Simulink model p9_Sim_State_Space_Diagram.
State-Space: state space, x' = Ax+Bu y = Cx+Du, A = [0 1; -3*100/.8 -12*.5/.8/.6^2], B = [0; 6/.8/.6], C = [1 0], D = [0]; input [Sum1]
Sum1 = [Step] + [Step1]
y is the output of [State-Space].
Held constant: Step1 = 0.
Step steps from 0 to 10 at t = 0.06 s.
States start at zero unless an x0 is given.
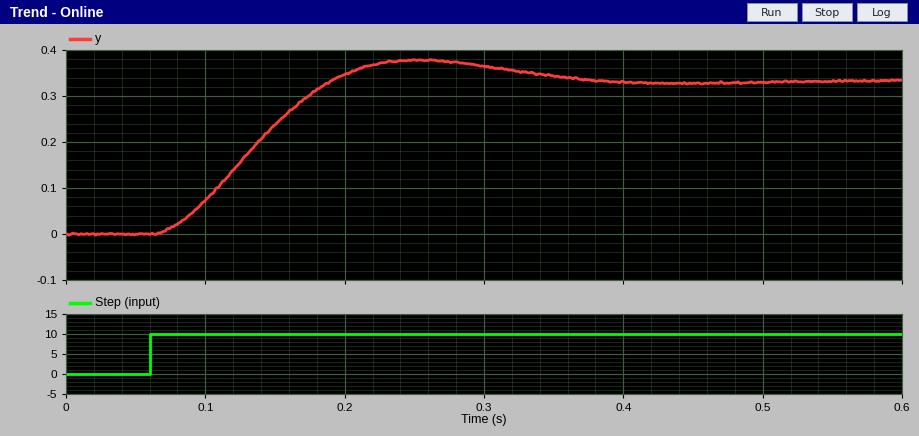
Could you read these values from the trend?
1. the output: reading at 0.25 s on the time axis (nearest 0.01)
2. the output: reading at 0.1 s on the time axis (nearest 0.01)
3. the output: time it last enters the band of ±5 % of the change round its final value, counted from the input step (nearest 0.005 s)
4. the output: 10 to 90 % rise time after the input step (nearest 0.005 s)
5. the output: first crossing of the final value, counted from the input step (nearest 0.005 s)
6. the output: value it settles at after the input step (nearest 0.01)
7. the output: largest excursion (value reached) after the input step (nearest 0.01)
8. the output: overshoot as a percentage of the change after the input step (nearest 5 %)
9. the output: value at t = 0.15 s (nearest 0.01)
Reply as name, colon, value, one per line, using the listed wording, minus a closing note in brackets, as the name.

the output: reading at 0.25 s on the time axis: 0.38
the output: reading at 0.1 s on the time axis: 0.07
the output: time it last enters the band of ±5 % of the change round its final value, counted from the input step: 0.275 s
the output: 10 to 90 % rise time after the input step: 0.090 s
the output: first crossing of the final value, counted from the input step: 0.130 s
the output: value it settles at after the input step: 0.33
the output: largest excursion (value reached) after the input step: 0.38
the output: overshoot as a percentage of the change after the input step: 15 %
the output: value at t = 0.15 s: 0.24
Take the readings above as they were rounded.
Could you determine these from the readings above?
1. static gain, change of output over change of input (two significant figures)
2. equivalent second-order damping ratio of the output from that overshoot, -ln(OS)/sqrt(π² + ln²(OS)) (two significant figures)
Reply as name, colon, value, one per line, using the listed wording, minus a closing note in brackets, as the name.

static gain, change of output over change of input: 0.033
equivalent second-order damping ratio of the output from that overshoot, -ln(OS)/sqrt(π² + ln²(OS)): 0.52
